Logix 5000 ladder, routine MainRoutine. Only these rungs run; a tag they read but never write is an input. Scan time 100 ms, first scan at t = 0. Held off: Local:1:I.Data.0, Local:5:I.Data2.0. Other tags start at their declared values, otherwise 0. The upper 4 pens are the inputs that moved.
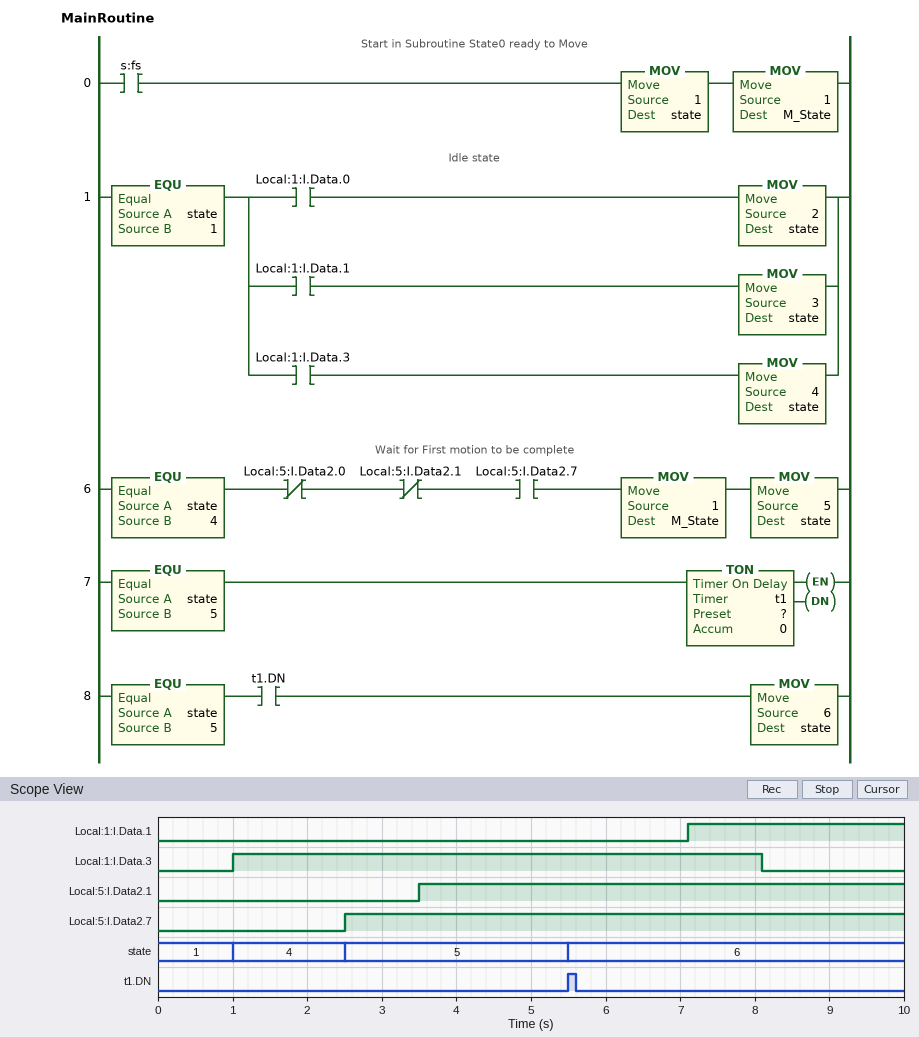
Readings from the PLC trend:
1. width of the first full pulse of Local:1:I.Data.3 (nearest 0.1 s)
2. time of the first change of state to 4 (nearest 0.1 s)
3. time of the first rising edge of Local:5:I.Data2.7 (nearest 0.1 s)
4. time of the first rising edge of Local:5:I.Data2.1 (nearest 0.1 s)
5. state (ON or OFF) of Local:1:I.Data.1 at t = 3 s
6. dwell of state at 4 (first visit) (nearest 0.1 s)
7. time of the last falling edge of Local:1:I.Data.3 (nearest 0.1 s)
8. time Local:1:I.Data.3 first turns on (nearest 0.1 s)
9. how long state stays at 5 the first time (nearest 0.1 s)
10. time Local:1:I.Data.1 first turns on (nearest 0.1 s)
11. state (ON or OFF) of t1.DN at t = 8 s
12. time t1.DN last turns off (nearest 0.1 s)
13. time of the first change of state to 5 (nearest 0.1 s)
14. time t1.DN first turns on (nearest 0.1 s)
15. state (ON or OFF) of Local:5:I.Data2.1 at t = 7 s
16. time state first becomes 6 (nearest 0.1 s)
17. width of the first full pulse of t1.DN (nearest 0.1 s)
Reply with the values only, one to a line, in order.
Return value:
7.1 s
1.0 s
2.5 s
3.5 s
OFF
1.5 s
8.1 s
1.0 s
3.0 s
7.1 s
OFF
5.6 s
2.5 s
5.5 s
ON
5.5 s
0.1 s
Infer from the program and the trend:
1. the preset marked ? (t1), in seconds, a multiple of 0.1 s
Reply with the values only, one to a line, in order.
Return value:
3.0 s
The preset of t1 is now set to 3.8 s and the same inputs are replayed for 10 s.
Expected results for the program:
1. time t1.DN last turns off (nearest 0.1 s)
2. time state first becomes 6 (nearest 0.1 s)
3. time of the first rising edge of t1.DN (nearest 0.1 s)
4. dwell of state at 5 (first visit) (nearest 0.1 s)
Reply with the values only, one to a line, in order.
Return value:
6.4 s
6.3 s
6.3 s
3.8 s
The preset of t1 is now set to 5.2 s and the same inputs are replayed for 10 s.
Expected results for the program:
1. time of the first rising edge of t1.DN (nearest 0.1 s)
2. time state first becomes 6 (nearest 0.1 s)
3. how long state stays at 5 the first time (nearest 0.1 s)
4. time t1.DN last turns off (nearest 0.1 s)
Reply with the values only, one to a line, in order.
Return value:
7.7 s
7.7 s
5.2 s
7.8 s
